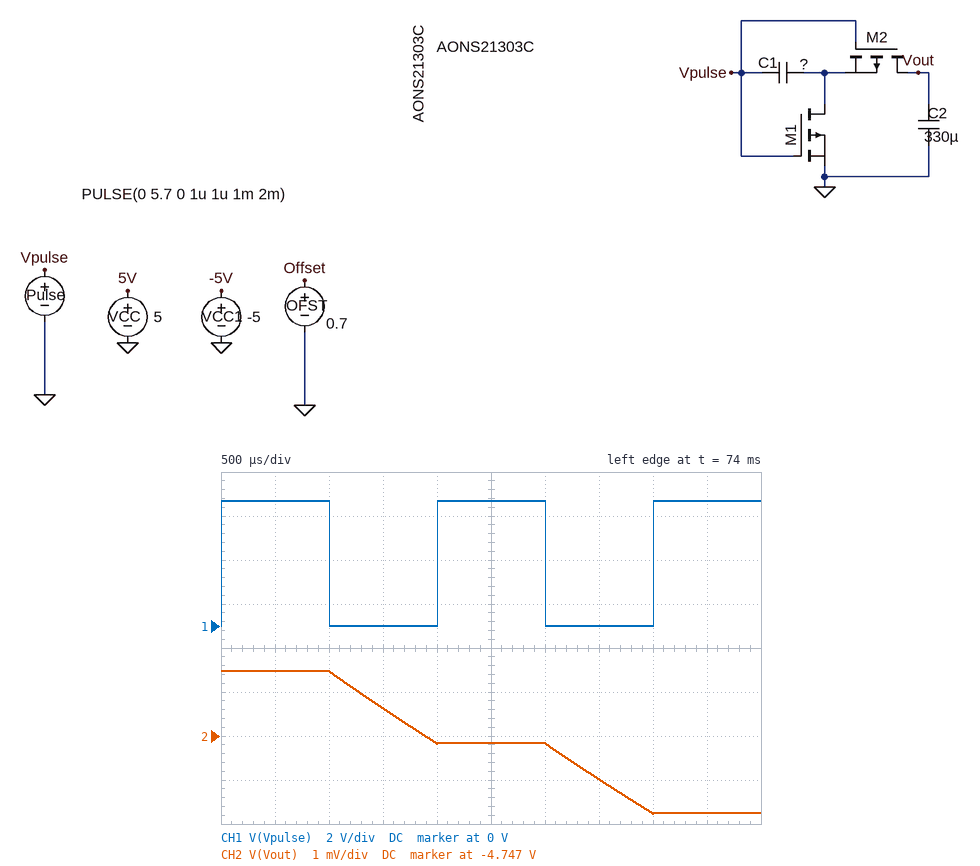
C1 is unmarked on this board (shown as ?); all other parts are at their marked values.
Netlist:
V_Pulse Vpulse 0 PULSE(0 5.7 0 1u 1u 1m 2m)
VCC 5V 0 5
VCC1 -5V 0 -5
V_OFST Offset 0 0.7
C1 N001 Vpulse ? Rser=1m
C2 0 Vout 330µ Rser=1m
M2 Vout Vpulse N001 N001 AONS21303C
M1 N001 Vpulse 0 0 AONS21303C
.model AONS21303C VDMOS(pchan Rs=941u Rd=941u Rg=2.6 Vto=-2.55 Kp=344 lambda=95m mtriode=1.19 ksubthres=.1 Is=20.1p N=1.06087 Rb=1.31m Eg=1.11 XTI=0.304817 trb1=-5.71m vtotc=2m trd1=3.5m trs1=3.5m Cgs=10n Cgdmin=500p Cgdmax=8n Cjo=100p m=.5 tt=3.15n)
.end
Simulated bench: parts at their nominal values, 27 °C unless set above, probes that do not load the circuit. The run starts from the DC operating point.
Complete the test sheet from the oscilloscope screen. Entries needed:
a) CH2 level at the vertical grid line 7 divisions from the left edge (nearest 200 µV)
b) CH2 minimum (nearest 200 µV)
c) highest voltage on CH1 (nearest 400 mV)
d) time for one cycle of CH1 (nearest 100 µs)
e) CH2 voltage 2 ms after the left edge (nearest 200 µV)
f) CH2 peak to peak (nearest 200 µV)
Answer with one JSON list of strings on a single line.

["-4.7480 V", "-4.7488 V", "5.6 V", "2.0 ms", "-4.7472 V", "3.2 mV"]
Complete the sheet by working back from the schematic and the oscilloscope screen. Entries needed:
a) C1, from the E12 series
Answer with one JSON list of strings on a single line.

["470 µF"]
